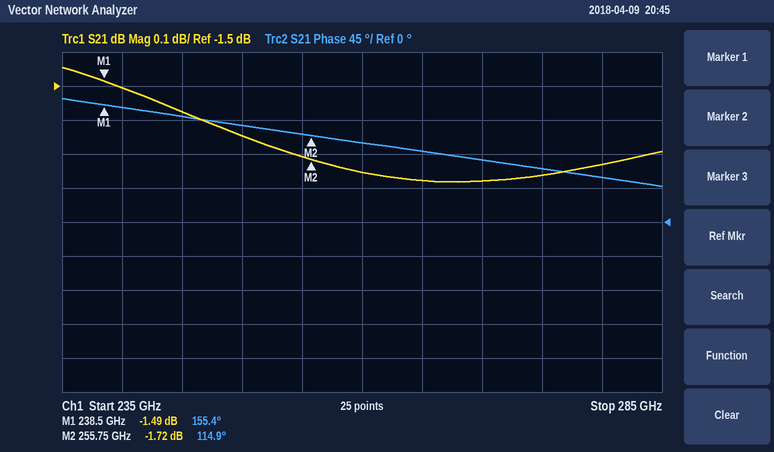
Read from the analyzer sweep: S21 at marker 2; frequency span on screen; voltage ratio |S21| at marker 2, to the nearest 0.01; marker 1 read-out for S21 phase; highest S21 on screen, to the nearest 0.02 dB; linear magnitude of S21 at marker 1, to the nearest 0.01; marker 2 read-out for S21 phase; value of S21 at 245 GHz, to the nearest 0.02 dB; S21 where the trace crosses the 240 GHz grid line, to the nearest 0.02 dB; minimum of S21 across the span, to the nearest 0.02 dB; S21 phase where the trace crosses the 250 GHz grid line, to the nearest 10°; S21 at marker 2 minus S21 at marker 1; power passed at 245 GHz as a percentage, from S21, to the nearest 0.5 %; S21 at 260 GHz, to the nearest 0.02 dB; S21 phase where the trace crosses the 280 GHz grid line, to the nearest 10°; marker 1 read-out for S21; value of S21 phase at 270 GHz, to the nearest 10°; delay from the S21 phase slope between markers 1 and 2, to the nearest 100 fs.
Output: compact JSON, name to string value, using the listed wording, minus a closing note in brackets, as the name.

{"S21 at marker 2": "-1.72 dB", "frequency span on screen": "50 GHz", "voltage ratio |S21| at marker 2, to the nearest 0.01": "0.82", "marker 1 read-out for S21 phase": "155.4°", "highest S21 on screen, to the nearest 0.02 dB": "-1.44 dB", "linear magnitude of S21 at marker 1, to the nearest 0.01": "0.84", "marker 2 read-out for S21 phase": "114.9°", "value of S21 at 245 GHz, to the nearest 0.02 dB": "-1.58 dB", "S21 where the trace crosses the 240 GHz grid line, to the nearest 0.02 dB": "-1.50 dB", "minimum of S21 across the span, to the nearest 0.02 dB": "-1.78 dB", "S21 phase where the trace crosses the 250 GHz grid line, to the nearest 10°": "130°", "S21 at marker 2 minus S21 at marker 1": "-0.23 dB", "power passed at 245 GHz as a percentage, from S21, to the nearest 0.5 %": "69.5 %", "S21 at 260 GHz, to the nearest 0.02 dB": "-1.76 dB", "S21 phase where the trace crosses the 280 GHz grid line, to the nearest 10°": "60°", "marker 1 read-out for S21": "-1.49 dB", "value of S21 phase at 270 GHz, to the nearest 10°": "80°", "delay from the S21 phase slope between markers 1 and 2, to the nearest 100 fs": "6.5 ps"}
